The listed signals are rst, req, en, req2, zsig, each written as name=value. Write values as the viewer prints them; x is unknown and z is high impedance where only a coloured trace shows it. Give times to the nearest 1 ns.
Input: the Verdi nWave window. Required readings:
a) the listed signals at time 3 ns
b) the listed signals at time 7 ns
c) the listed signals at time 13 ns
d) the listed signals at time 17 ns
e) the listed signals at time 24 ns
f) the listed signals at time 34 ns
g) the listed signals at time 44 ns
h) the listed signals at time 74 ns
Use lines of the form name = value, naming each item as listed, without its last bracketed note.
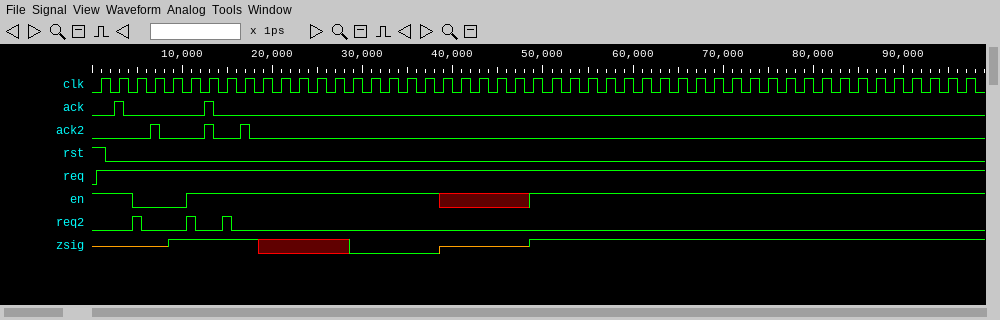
the listed signals at time 3 ns = rst=0, req=1, en=1, req2=0, zsig=z
the listed signals at time 7 ns = rst=0, req=1, en=0, req2=0, zsig=z
the listed signals at time 13 ns = rst=0, req=1, en=1, req2=0, zsig=1
the listed signals at time 17 ns = rst=0, req=1, en=1, req2=0, zsig=1
the listed signals at time 24 ns = rst=0, req=1, en=1, req2=0, zsig=x
the listed signals at time 34 ns = rst=0, req=1, en=1, req2=0, zsig=0
the listed signals at time 44 ns = rst=0, req=1, en=x, req2=0, zsig=z
the listed signals at time 74 ns = rst=0, req=1, en=1, req2=0, zsig=1
